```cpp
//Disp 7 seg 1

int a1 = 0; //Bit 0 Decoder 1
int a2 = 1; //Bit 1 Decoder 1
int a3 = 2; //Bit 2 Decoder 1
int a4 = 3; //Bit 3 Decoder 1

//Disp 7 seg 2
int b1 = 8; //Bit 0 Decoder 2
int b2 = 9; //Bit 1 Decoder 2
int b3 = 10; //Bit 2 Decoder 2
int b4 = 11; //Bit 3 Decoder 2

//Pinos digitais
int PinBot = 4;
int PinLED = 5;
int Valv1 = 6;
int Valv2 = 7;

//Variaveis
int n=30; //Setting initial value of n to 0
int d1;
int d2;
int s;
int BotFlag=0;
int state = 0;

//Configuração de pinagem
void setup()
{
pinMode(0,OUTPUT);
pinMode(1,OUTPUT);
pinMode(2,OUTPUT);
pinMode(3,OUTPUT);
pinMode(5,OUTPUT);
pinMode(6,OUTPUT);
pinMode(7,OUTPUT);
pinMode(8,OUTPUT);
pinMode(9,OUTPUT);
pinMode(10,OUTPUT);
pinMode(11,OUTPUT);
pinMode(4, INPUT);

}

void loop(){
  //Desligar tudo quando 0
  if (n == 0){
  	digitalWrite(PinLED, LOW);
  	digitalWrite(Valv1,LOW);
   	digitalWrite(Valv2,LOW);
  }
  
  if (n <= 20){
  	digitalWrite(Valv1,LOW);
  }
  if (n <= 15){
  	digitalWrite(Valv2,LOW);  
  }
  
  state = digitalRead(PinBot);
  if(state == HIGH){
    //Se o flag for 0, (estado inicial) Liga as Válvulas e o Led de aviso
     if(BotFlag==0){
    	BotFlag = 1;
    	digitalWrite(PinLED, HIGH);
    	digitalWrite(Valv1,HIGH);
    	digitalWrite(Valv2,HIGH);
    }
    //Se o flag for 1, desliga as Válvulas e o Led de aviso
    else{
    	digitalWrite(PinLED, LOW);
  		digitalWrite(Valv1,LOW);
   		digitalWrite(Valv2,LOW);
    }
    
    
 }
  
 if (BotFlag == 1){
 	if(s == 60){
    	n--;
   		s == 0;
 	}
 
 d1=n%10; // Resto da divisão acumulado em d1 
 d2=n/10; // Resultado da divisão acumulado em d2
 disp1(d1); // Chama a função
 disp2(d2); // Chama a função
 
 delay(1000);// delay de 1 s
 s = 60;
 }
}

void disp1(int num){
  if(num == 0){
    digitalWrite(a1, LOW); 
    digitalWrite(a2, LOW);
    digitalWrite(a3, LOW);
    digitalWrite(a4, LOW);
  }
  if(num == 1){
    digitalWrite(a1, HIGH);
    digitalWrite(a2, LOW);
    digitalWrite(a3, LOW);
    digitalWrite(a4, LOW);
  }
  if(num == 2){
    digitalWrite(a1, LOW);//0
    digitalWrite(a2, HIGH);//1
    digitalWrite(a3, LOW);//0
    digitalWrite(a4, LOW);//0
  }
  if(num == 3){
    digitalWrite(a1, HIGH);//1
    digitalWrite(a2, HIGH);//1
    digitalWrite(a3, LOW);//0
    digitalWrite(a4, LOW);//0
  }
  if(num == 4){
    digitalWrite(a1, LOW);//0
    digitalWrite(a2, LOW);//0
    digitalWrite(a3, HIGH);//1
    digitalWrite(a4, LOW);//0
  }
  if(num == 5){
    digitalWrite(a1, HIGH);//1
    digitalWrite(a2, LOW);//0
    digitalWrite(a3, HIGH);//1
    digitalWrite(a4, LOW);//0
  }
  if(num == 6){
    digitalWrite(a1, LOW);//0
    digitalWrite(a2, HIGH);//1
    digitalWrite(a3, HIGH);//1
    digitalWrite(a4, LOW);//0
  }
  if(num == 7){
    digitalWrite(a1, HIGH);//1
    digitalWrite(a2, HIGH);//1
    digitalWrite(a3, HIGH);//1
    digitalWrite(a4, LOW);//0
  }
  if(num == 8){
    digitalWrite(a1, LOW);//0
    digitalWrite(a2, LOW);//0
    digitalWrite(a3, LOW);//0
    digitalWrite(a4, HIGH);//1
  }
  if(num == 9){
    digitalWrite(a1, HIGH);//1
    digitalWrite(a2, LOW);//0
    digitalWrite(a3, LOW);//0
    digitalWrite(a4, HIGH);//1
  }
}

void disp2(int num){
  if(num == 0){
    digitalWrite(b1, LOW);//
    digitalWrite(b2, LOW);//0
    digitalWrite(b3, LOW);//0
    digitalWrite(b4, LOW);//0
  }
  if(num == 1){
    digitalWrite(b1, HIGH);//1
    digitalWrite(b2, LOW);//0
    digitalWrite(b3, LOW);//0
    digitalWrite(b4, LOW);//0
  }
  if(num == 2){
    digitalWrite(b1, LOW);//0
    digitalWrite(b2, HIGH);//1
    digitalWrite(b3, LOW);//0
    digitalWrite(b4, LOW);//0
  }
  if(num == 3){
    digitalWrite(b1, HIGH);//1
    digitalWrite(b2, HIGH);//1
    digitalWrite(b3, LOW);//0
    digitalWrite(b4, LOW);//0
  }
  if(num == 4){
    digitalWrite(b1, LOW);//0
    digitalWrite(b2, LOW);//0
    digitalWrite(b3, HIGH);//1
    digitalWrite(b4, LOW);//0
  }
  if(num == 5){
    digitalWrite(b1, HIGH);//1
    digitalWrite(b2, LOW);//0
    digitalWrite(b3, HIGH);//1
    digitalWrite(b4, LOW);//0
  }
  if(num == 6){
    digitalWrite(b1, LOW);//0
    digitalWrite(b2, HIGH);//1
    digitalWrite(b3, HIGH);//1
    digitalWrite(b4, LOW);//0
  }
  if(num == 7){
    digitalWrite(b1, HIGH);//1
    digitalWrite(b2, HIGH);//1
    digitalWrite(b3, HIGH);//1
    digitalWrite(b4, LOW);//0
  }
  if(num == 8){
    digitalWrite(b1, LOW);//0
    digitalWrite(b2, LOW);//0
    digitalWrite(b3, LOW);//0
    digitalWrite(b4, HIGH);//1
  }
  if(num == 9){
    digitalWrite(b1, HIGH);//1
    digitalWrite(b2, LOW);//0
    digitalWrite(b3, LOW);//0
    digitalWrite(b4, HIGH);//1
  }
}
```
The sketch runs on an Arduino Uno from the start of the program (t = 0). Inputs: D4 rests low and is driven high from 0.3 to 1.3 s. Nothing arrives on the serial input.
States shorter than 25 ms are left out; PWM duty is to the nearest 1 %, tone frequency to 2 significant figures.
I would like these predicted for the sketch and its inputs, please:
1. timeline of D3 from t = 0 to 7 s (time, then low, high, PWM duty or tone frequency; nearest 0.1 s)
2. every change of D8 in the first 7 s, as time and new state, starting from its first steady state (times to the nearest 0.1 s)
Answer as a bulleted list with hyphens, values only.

- 0 s low; 1.3 s high; 3.3 s low
- 0 s low; 0.3 s high; 1.3 s low
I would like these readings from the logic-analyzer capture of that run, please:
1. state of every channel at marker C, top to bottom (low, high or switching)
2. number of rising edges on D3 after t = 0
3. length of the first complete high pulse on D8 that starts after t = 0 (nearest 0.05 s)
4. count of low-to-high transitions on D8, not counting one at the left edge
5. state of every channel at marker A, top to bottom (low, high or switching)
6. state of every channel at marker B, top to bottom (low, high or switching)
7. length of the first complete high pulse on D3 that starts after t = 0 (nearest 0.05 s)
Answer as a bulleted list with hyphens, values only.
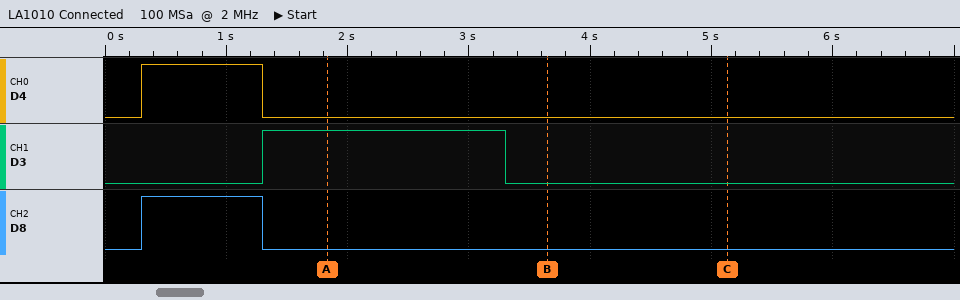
- D4 low, D3 low, D8 low
- 1
- 1.00 s
- 1
- D4 low, D3 high, D8 low
- D4 low, D3 low, D8 low
- 2.00 s
